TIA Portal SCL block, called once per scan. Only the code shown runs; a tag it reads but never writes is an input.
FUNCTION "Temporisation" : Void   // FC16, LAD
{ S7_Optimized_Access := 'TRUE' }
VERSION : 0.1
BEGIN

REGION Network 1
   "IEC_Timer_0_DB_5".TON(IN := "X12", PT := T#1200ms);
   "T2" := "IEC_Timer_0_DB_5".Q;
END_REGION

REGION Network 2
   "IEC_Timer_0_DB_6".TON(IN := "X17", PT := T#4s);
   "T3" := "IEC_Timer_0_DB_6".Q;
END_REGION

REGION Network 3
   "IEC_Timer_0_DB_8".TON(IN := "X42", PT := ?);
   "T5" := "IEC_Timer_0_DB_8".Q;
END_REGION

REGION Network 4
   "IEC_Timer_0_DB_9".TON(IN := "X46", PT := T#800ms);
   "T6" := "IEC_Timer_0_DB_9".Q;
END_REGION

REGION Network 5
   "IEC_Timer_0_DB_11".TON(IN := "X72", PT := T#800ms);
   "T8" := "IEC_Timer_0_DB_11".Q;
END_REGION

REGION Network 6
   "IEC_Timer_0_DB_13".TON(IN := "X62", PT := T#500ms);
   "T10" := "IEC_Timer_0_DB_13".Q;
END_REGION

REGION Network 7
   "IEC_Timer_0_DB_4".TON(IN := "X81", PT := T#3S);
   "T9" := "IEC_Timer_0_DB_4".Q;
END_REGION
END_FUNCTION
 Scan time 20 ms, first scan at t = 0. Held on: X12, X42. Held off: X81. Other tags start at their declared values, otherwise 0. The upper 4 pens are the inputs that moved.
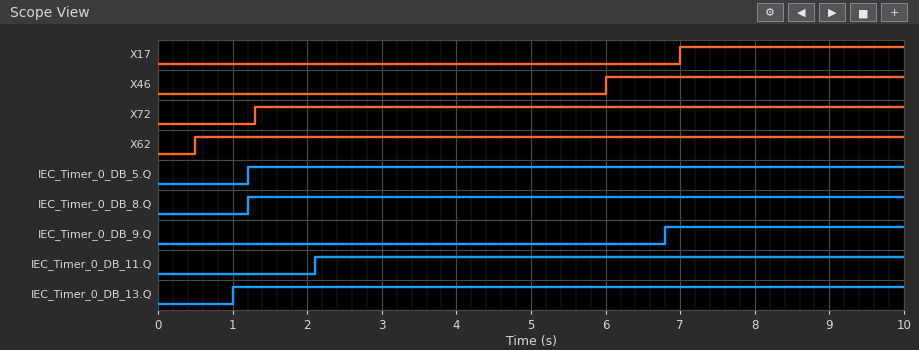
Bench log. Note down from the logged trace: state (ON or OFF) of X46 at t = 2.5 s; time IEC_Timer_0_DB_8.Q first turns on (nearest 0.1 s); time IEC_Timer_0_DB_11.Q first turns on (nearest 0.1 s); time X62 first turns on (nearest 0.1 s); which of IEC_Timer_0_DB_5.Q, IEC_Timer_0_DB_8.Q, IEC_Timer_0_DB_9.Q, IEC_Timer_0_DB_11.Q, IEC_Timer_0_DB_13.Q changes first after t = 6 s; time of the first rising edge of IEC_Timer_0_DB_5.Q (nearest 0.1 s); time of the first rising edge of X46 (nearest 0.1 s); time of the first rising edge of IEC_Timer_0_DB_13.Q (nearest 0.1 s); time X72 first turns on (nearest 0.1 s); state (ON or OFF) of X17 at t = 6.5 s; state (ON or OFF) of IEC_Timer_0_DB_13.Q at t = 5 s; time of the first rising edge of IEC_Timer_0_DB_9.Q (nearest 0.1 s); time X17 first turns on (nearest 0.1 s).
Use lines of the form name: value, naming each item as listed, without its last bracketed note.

state (ON or OFF) of X46 at t = 2.5 s: OFF
time IEC_Timer_0_DB_8.Q first turns on: 1.2 s
time IEC_Timer_0_DB_11.Q first turns on: 2.1 s
time X62 first turns on: 0.5 s
which of IEC_Timer_0_DB_5.Q, IEC_Timer_0_DB_8.Q, IEC_Timer_0_DB_9.Q, IEC_Timer_0_DB_11.Q, IEC_Timer_0_DB_13.Q changes first after t = 6 s: IEC_Timer_0_DB_9.Q
time of the first rising edge of IEC_Timer_0_DB_5.Q: 1.2 s
time of the first rising edge of X46: 6.0 s
time of the first rising edge of IEC_Timer_0_DB_13.Q: 1.0 s
time X72 first turns on: 1.3 s
state (ON or OFF) of X17 at t = 6.5 s: OFF
state (ON or OFF) of IEC_Timer_0_DB_13.Q at t = 5 s: ON
time of the first rising edge of IEC_Timer_0_DB_9.Q: 6.8 s
time X17 first turns on: 7.0 s
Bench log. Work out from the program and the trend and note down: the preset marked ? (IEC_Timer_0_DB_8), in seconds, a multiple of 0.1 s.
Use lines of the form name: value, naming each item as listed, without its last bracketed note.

the preset marked ? (IEC_Timer_0_DB_8), in seconds, a multiple of 0.1 s: 1.2 s
